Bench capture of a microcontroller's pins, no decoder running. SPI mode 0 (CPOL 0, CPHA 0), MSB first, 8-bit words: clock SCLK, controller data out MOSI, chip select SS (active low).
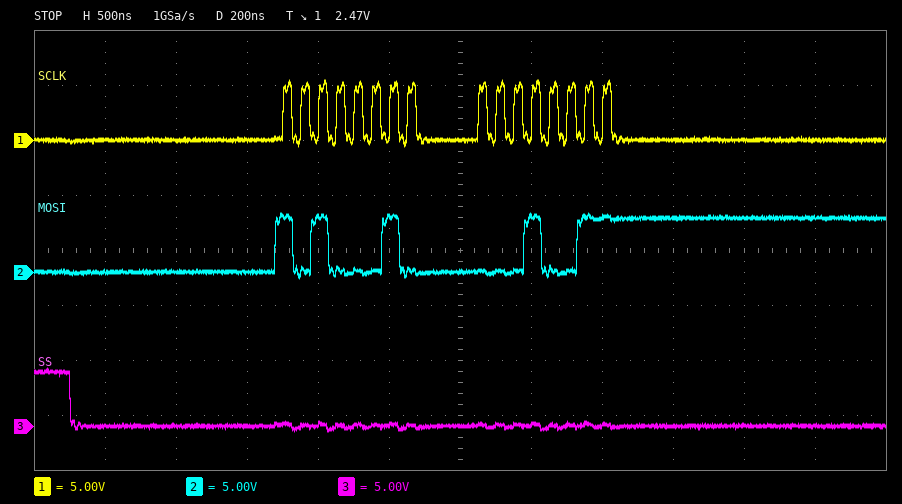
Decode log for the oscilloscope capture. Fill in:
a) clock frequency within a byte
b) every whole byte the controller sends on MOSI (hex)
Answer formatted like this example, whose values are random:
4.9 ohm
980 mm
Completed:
8 MHz
A2 13
